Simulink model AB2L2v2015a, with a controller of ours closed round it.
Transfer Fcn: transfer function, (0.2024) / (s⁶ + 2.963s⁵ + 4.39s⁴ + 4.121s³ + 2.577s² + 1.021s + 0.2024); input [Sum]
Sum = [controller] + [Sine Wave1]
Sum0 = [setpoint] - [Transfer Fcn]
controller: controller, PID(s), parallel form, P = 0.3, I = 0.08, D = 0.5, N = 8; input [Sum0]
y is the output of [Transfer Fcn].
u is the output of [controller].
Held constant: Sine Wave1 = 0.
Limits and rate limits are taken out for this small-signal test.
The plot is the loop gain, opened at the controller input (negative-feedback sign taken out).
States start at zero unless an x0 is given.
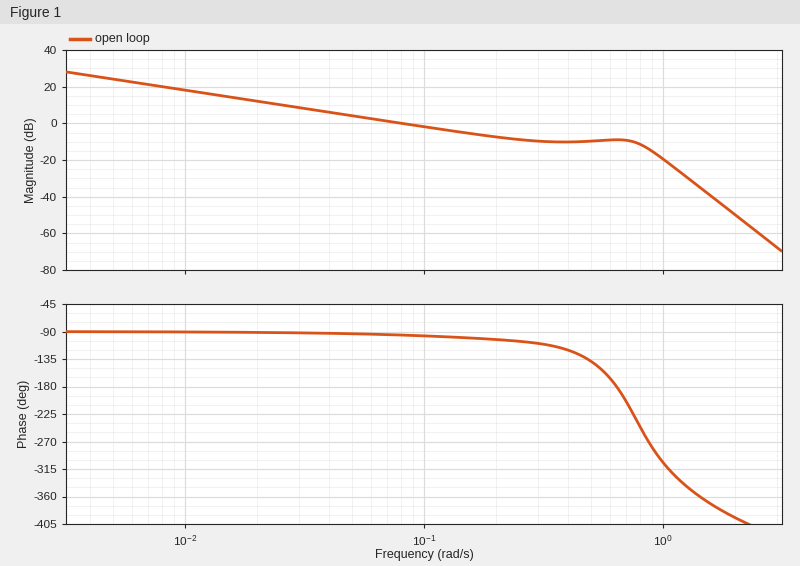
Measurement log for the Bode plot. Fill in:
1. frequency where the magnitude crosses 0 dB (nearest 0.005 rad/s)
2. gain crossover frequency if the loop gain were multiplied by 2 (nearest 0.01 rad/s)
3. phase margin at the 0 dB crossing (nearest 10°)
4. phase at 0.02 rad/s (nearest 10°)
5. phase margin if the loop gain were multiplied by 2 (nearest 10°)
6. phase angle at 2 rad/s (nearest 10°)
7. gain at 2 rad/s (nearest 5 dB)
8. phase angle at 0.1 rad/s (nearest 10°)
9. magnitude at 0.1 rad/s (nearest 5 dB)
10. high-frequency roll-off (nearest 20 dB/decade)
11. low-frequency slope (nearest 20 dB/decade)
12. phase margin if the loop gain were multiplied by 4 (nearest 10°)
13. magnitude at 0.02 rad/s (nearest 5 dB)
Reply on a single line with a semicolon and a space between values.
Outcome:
0.080 rad/s; 0.17 rad/s; 80°; -90°; 80°; -390°; -50 dB; -100°; 0 dB; -100 dB/decade; -20 dB/decade; -70°; 10 dB
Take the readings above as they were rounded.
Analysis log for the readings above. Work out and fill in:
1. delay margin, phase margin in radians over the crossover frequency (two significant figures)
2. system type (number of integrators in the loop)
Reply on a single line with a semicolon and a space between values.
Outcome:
17 s; 1
